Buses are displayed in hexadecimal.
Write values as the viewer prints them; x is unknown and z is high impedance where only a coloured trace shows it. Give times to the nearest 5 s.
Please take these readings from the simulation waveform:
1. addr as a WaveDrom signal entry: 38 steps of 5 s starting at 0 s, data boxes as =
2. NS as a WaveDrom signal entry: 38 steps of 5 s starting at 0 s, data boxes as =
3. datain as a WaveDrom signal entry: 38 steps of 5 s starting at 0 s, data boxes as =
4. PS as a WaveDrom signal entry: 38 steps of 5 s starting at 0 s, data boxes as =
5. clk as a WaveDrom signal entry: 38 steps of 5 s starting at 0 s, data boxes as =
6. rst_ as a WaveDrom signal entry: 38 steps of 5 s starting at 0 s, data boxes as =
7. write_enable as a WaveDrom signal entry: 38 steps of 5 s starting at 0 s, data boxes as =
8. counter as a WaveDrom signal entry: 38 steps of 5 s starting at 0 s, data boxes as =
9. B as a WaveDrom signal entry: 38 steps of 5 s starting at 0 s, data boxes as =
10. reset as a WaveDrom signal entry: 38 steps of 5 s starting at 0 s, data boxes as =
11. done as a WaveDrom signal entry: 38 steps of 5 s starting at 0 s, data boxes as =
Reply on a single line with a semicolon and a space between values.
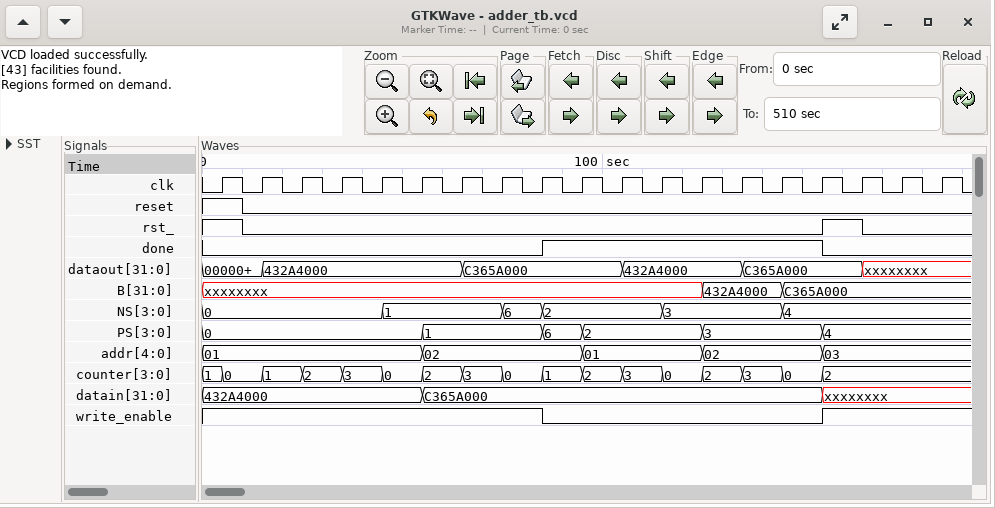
{name: 'addr', wave: '=..........=.......=.....=.....=......', data: '01 02 01 02 03'}; {name: 'NS', wave: '=........=.....=.=.....=.....=........', data: '0 1 6 2 3 4'}; {name: 'datain', wave: '=..........=...................x......', data: '432A4000 C365A000'}; {name: 'PS', wave: '=..........=.....=.=.....=.....=......', data: '0 1 6 2 3 4'}; {name: 'clk', wave: '01010101010101010101010101010101010101'}; {name: 'rst_', wave: '1.0............................1.0....'}; {name: 'write_enable', wave: '1................0.............1......'}; {name: 'counter', wave: '==.=.=.=.=.=.=.=.=.=.=.=.=.=.=.=......', data: '1 0 1 2 3 0 2 3 0 1 2 3 0 2 3 0 2'}; {name: 'B', wave: 'x........................=...=........', data: '432A4000 C365A000'}; {name: 'reset', wave: '1.0...................................'}; {name: 'done', wave: '0................1.............0......'}
